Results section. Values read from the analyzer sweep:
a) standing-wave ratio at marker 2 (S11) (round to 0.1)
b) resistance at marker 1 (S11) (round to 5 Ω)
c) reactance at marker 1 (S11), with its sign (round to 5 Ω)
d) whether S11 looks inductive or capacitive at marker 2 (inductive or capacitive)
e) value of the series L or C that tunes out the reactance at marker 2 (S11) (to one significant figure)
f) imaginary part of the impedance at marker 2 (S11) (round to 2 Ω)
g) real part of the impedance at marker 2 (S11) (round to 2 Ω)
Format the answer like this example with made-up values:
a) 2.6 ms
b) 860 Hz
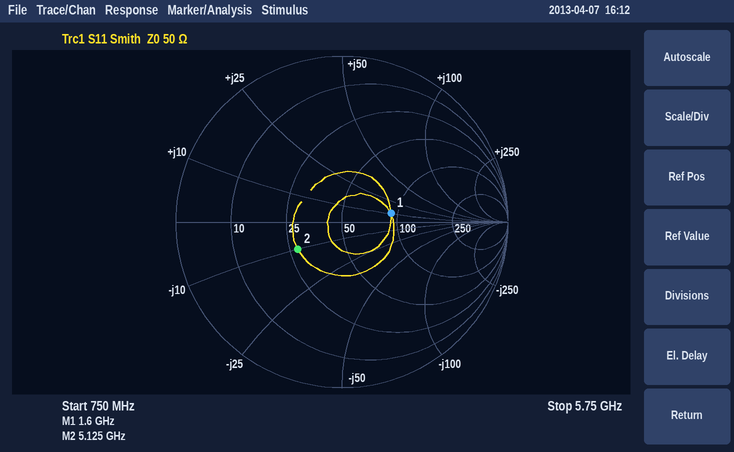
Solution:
a) 1.9
b) 90 Ω
c) +10 Ω
d) capacitive
e) 300 pH
f) -10 Ω
g) 28 Ω
